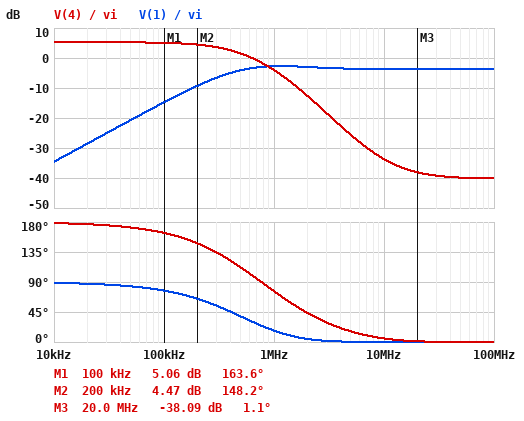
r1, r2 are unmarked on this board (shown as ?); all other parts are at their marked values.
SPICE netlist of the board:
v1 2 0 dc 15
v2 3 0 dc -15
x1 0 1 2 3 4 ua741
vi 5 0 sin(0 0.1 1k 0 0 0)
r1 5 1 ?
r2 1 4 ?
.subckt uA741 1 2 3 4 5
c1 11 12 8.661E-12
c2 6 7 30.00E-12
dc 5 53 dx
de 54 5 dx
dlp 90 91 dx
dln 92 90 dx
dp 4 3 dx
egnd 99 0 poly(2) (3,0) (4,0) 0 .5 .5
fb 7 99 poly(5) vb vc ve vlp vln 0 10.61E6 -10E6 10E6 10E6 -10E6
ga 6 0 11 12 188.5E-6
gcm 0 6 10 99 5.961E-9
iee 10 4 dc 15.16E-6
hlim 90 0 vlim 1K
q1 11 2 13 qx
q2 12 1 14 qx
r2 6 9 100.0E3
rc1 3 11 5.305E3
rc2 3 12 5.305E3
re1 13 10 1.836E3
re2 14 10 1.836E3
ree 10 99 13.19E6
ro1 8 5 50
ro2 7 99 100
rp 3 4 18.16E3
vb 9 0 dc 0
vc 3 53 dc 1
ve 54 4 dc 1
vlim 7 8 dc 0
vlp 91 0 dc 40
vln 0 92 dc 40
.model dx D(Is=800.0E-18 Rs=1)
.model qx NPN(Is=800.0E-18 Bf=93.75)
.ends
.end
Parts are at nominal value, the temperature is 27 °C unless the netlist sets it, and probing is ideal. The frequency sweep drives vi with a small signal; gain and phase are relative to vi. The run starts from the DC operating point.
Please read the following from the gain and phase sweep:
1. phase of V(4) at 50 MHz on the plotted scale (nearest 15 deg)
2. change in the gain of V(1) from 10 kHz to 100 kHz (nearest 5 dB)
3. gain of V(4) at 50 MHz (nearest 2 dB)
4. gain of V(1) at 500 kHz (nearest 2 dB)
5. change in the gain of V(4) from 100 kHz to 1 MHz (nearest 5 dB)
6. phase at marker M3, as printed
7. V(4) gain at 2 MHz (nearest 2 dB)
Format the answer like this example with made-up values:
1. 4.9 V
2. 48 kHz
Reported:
1. 0 deg
2. 20 dB
3. -40 dB
4. -4 dB
5. -10 dB
6. 1.1 deg
7. -12 dB
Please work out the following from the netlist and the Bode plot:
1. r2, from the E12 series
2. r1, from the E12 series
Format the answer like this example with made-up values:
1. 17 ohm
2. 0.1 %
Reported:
1. 3.3 kΩ
2. 1.8 kΩ
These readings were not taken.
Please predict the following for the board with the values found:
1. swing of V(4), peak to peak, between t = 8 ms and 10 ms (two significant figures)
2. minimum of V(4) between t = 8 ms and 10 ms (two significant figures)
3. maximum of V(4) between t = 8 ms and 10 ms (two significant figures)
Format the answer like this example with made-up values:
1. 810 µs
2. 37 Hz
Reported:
1. 370 mV
2. -180 mV
3. 180 mV
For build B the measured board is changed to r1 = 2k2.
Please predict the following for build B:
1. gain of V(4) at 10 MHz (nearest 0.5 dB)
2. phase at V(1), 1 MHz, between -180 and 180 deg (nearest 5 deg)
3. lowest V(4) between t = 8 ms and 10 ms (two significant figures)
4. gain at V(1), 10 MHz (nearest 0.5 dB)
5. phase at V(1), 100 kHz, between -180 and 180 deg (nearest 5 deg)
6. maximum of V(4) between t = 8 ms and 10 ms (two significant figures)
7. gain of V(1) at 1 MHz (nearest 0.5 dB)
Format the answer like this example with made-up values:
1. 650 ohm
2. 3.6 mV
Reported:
1. -34.5 dB
2. 20 deg
3. -150 mV
4. -4.5 dB
5. 80 deg
6. 150 mV
7. -3.5 dB
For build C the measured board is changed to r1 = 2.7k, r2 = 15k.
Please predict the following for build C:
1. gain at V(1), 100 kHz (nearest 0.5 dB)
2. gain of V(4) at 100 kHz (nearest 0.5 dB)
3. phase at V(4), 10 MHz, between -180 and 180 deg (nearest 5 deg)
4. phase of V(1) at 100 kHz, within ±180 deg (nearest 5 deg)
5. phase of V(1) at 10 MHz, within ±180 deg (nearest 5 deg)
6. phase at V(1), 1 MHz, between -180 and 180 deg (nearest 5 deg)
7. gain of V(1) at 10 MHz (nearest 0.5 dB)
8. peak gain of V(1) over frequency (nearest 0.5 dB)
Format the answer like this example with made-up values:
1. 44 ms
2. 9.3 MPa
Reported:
1. -6.5 dB
2. 13.5 dB
3. 10 deg
4. 60 deg
5. 0 deg
6. 5 deg
7. -1.5 dB
8. -1.0 dB
